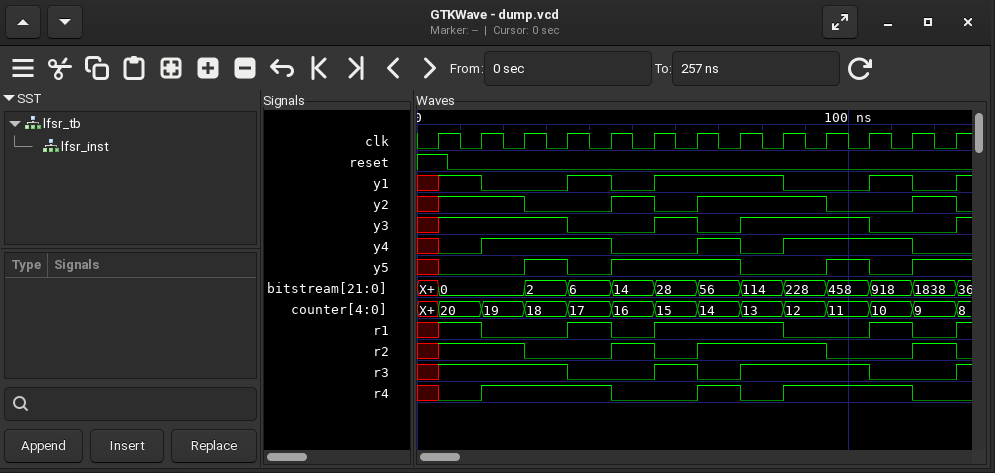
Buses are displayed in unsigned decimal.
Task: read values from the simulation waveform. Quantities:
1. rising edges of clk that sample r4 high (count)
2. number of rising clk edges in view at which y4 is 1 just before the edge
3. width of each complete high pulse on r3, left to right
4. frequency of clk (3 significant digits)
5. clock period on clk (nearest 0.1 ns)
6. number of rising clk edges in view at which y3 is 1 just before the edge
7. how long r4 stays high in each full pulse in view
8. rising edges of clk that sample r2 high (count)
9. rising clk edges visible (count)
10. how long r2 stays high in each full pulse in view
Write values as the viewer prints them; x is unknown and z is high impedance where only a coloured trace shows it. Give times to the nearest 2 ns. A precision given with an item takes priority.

7
7
10 ns, 30 ns
100 MHz
10 ns
7
30 ns, 10 ns, 30 ns
7
13
10 ns, 30 ns, 10 ns
